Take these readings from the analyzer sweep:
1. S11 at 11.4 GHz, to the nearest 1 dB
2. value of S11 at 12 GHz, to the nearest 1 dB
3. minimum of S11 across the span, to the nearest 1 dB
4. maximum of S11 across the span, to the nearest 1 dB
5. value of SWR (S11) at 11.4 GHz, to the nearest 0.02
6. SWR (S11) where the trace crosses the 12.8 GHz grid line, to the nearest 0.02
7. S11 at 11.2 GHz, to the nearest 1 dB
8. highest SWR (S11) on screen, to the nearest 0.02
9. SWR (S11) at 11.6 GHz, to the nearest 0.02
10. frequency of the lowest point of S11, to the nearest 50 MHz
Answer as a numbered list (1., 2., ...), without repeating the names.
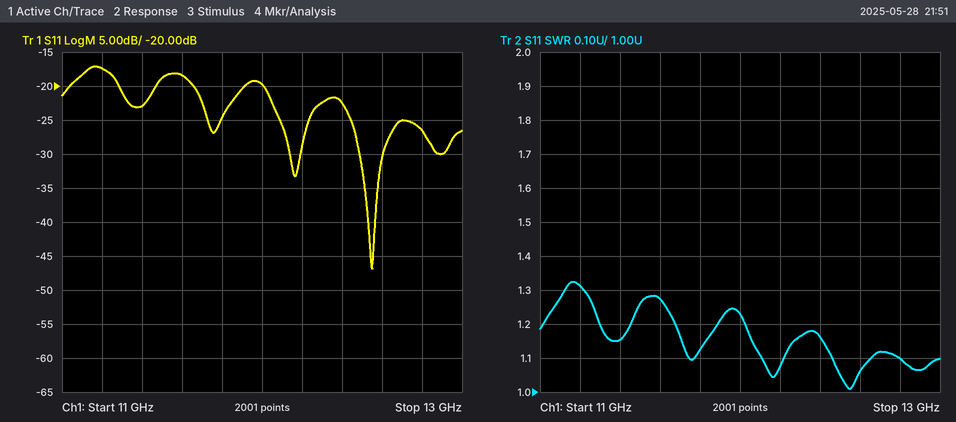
1. -23 dB
2. -20 dB
3. -47 dB
4. -17 dB
5. 1.16
6. 1.10
7. -17 dB
8. 1.32
9. 1.28
10. 12.55 GHz
